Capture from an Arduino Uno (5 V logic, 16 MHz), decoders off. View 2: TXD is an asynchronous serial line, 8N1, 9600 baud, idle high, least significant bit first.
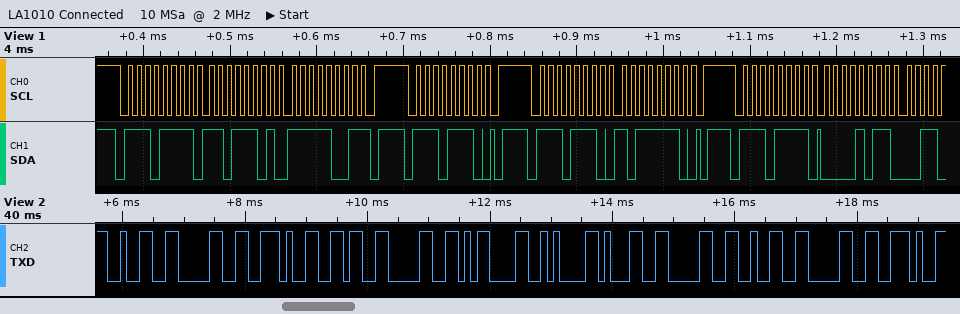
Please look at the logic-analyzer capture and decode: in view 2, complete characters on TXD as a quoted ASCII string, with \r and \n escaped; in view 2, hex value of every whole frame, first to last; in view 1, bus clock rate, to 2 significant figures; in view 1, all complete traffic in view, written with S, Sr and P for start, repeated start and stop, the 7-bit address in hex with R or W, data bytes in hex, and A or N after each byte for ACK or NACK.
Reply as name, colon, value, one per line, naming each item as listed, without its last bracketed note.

in view 2, complete characters on TXD as a quoted ASCII string, with \r and \n escaped: "20.60\r\n1020."
in view 2, hex value of every whole frame, first to last: 32 30 2E 36 30 0D 0A 31 30 32 30 2E
in view 1, bus clock rate, to 2 significant figures: 100 kHz
in view 1, all complete traffic in view, written with S, Sr and P for start, repeated start and stop, the 7-bit address in hex with R or W, data bytes in hex, and A or N after each byte for ACK or NACK: S 77R A DD A F9 N P S 77W A P S 77W A BE A P S 77R A 0B A
